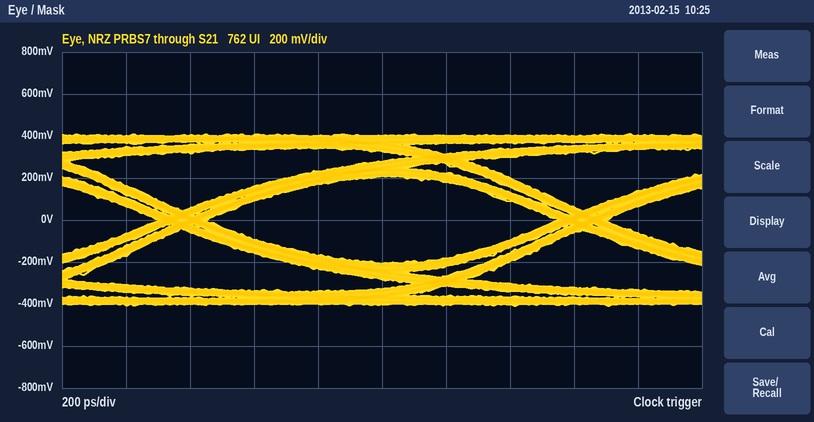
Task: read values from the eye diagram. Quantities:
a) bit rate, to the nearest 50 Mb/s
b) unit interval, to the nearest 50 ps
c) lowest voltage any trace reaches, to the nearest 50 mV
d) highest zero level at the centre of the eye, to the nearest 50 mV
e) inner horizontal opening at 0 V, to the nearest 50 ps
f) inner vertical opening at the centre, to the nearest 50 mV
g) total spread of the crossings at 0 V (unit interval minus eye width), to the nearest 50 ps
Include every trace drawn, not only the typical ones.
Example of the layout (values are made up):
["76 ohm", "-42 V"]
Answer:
["800 Mb/s", "1.25 ns", "-400 mV", "-200 mV", "1.10 ns", "400 mV", "150 ps"]
